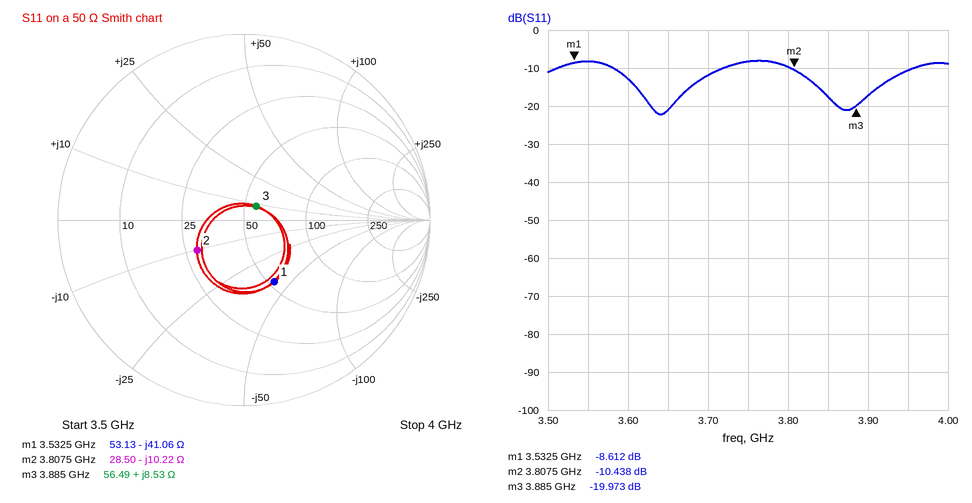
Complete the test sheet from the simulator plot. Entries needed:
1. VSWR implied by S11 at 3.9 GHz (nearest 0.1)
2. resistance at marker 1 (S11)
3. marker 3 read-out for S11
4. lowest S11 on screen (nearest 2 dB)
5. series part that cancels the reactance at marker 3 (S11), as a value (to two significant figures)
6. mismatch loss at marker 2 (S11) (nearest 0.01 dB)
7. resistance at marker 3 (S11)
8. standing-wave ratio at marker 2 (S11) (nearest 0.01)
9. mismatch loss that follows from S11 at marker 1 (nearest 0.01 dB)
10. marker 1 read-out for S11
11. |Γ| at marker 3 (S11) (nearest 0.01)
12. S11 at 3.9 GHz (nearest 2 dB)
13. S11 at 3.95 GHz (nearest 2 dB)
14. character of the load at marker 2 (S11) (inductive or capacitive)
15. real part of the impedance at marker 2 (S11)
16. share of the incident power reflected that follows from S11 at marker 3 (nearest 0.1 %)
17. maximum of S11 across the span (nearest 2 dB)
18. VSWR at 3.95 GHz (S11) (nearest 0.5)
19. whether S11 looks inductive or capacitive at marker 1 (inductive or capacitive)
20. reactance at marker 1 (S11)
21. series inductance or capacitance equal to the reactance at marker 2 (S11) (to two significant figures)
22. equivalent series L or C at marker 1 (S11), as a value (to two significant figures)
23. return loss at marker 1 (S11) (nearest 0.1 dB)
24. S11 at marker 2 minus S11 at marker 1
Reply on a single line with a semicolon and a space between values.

1.3; 53.13 Ω; -19.973 dB; -22 dB; 4.8 pF; 0.41 dB; 56.49 Ω; 1.86; 0.64 dB; -8.612 dB; 0.10; -18 dB; -10 dB; capacitive; 28.50 Ω; 1.0 %; -8 dB; 2.0; capacitive; -41.06 Ω; 4.1 pF; 1.1 pF; 8.6 dB; -1.826 dB
